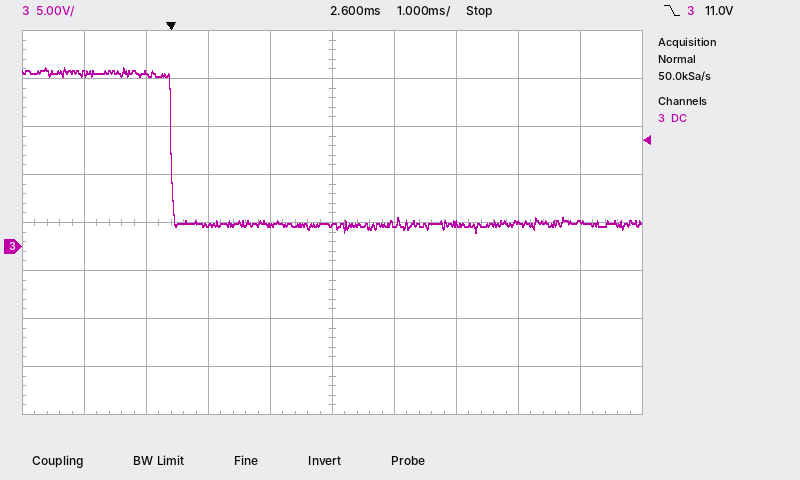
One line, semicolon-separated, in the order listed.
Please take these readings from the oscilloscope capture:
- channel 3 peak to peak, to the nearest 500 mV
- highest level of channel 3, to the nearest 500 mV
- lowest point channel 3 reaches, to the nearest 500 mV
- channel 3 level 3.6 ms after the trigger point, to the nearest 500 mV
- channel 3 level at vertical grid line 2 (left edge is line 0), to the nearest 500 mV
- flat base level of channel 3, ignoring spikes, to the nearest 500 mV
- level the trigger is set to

17.0 V; 18.5 V; 1.5 V; 2.5 V; 18.0 V; 2.5 V; 11.0 V
